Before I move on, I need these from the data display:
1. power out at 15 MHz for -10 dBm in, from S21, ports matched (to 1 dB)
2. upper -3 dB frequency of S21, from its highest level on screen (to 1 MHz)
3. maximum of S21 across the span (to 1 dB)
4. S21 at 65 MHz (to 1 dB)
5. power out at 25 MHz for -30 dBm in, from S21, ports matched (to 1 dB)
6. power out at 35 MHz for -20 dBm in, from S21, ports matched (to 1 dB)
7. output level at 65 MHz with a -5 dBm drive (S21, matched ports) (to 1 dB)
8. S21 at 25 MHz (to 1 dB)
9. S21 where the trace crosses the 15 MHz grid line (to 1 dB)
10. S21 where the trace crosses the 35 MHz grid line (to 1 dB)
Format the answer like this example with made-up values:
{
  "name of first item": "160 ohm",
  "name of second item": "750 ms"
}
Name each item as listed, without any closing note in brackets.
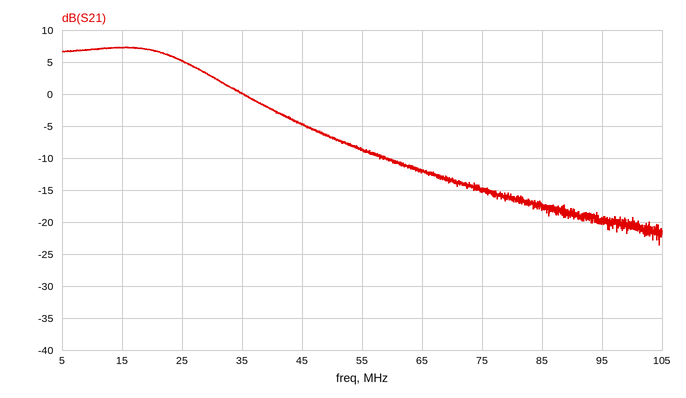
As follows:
{
  "power out at 15 MHz for -10 dBm in, from S21, ports matched": "-3 dBm",
  "upper -3 dB frequency of S21, from its highest level on screen": "27 MHz",
  "maximum of S21 across the span": "7 dB",
  "S21 at 65 MHz": "-12 dB",
  "power out at 25 MHz for -30 dBm in, from S21, ports matched": "-25 dBm",
  "power out at 35 MHz for -20 dBm in, from S21, ports matched": "-20 dBm",
  "output level at 65 MHz with a -5 dBm drive (S21, matched ports)": "-17 dBm",
  "S21 at 25 MHz": "5 dB",
  "S21 where the trace crosses the 15 MHz grid line": "7 dB",
  "S21 where the trace crosses the 35 MHz grid line": "0 dB"
}
